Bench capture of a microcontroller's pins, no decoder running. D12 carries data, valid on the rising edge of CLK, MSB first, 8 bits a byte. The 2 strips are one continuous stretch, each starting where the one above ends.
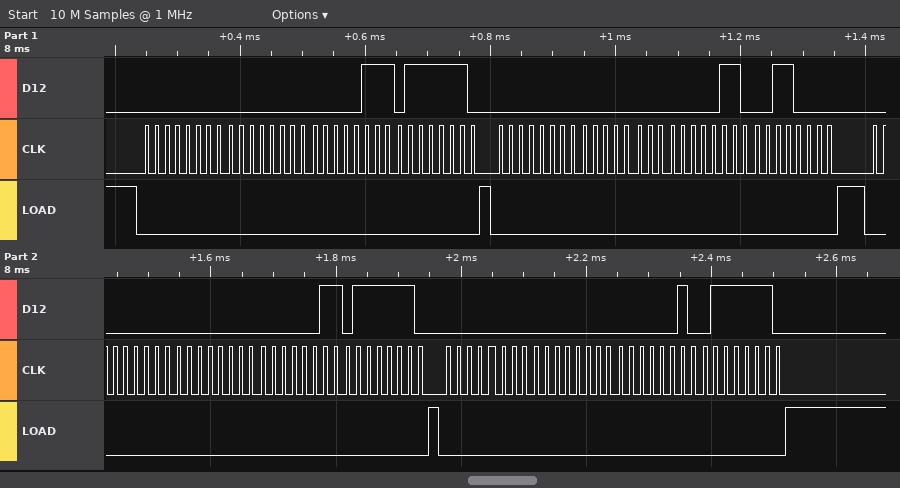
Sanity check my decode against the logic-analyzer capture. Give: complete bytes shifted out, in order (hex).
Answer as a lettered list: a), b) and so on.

a) 00 00 07 7E 00 00 06 30 00 00 03 7E 00 00 02 7E
